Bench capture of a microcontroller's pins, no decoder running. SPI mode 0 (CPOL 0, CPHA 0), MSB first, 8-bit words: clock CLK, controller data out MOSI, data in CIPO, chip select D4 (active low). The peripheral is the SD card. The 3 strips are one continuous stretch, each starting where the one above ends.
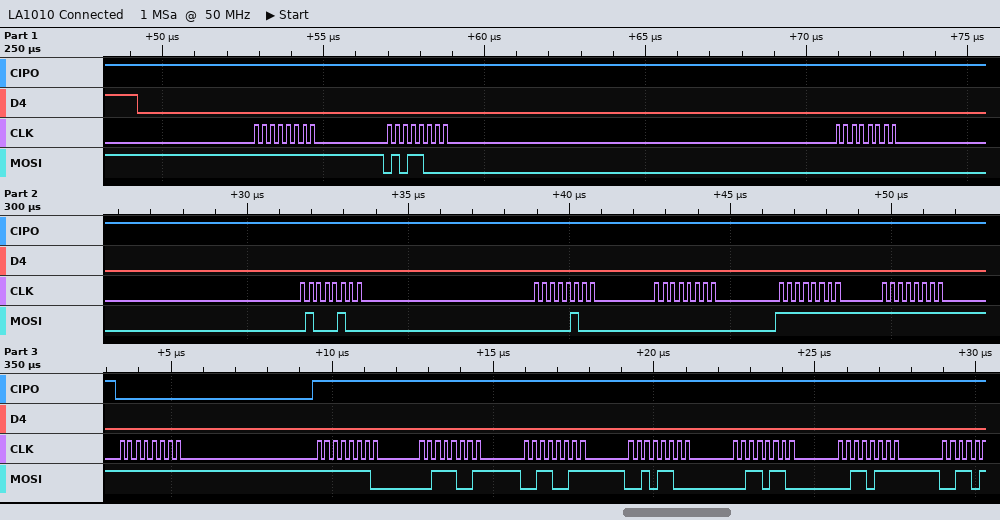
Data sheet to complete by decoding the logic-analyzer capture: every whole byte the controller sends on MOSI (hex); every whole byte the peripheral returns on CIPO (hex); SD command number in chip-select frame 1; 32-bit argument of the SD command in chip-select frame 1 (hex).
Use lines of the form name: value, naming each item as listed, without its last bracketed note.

every whole byte the controller sends on MOSI: 0xFF 0x58 0x00 0x44 0x04 0x00 0xFF 0xFF 0xFF 0xFE 0x39 0x33 0x2C 0x36 0x37
every whole byte the peripheral returns on CIPO: 0xFF 0xFF 0xFF 0xFF 0xFF 0xFF 0xFF 0xFF 0x00 0xFF 0xFF 0xFF 0xFF 0xFF 0xFF
SD command number in chip-select frame 1: CMD24
32-bit argument of the SD command in chip-select frame 1: 0x00440400
